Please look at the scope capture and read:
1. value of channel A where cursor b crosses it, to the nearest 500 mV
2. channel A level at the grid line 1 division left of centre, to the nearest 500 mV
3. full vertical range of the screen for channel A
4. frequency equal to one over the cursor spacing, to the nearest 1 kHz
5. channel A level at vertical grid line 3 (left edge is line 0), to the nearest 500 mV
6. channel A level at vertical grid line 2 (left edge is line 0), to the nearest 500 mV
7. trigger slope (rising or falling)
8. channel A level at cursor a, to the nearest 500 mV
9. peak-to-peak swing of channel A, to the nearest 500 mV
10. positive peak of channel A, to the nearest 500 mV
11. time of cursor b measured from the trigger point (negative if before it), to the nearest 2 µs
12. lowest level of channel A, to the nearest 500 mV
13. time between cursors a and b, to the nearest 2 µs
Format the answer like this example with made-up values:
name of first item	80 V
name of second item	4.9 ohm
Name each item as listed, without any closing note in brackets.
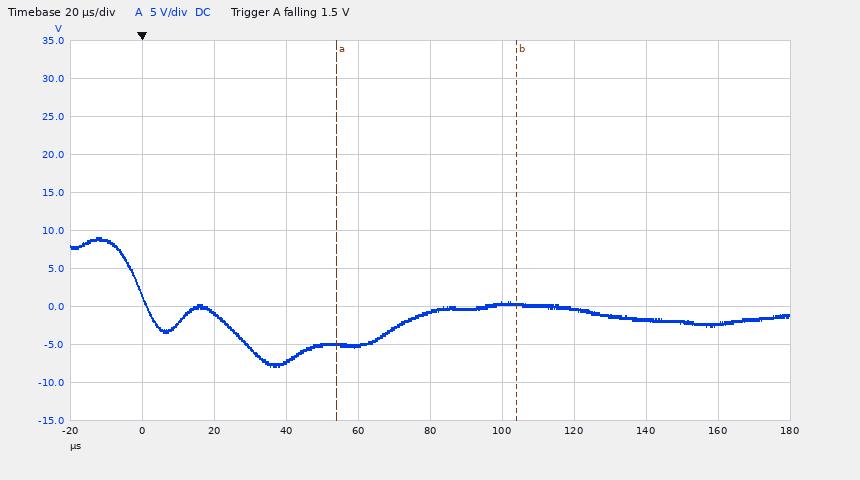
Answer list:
value of channel A where cursor b crosses it, to the nearest 500 mV	500 mV
channel A level at the grid line 1 division left of centre, to the nearest 500 mV	-5.0 V
full vertical range of the screen for channel A	50 V
frequency equal to one over the cursor spacing, to the nearest 1 kHz	20 kHz
channel A level at vertical grid line 3 (left edge is line 0), to the nearest 500 mV	-7.5 V
channel A level at vertical grid line 2 (left edge is line 0), to the nearest 500 mV	-1.0 V
trigger slope	falling
channel A level at cursor a, to the nearest 500 mV	-5.0 V
peak-to-peak swing of channel A, to the nearest 500 mV	17.0 V
positive peak of channel A, to the nearest 500 mV	9.0 V
time of cursor b measured from the trigger point (negative if before it), to the nearest 2 µs	+104 µs
lowest level of channel A, to the nearest 500 mV	-8.0 V
time between cursors a and b, to the nearest 2 µs	50 µs
